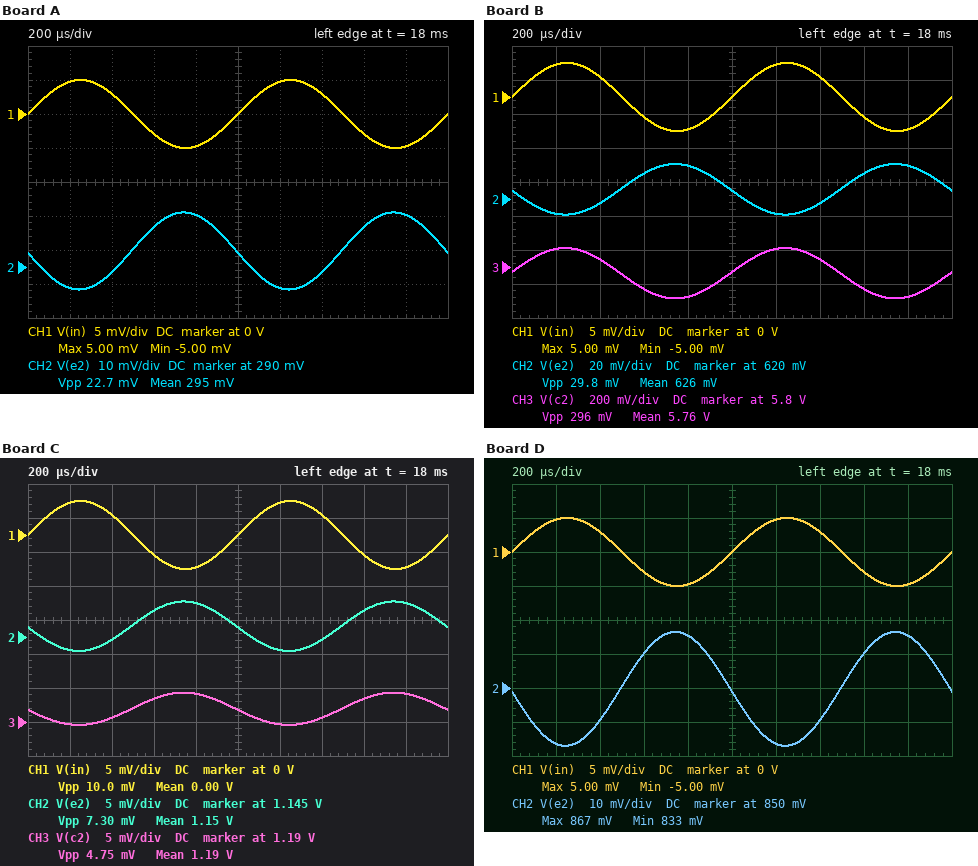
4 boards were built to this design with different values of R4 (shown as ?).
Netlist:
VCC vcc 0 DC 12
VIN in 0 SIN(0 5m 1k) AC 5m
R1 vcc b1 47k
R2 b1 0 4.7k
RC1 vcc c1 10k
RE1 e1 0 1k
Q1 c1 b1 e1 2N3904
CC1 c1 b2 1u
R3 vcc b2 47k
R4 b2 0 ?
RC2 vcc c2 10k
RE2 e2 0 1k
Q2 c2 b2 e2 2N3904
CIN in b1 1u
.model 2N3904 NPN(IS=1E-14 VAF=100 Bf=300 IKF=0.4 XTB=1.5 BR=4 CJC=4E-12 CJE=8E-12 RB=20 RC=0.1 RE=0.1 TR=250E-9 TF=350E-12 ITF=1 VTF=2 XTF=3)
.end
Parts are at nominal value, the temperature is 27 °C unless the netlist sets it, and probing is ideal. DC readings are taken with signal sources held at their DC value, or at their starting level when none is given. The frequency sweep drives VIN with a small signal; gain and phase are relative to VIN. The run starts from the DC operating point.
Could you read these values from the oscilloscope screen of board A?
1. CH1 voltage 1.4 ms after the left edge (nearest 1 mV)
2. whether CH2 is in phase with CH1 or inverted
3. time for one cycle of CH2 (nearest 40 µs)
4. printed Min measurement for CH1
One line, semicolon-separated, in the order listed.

3 mV; inverted; 1.00 ms; -5.00 mV
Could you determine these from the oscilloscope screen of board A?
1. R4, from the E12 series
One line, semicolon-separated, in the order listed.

3.9 kΩ
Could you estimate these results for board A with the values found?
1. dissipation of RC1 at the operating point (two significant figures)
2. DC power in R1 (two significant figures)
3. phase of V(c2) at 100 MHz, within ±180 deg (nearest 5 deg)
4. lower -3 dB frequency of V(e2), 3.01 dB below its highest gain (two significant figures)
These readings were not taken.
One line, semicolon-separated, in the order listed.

2.0 mW; 2.5 mW; 95 deg; 41 Hz
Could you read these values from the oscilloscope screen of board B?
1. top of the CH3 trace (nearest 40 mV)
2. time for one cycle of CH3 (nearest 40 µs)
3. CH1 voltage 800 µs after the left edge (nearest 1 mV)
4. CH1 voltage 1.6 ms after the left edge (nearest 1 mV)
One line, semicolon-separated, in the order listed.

5.92 V; 1.00 ms; -5 mV; -3 mV
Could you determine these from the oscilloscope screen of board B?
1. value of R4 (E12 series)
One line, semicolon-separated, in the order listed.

5.6 kΩ
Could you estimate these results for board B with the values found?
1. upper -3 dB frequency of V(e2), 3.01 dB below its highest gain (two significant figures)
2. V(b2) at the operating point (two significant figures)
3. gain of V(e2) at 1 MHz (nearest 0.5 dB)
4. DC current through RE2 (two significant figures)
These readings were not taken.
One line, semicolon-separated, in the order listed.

1.6 MHz; 1.3 V; 8.0 dB; 630 µA
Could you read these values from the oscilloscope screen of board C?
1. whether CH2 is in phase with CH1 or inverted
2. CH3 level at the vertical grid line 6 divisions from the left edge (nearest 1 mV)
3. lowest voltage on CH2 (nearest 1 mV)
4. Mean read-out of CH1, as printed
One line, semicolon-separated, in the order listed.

inverted; 1.190 V; 1.143 V; 0.00 V
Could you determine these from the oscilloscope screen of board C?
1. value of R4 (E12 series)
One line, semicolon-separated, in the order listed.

12 kΩ
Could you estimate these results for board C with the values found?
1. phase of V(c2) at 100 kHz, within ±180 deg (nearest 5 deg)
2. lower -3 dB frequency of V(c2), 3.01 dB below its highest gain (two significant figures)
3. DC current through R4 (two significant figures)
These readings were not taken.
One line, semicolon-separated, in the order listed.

-170 deg; 440 kHz; 150 µA
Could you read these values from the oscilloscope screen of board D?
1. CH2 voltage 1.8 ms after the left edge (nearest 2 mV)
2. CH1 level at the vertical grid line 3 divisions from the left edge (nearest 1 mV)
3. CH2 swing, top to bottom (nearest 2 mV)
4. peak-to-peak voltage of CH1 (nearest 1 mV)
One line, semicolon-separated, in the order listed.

866 mV; -3 mV; 34 mV; 10 mV
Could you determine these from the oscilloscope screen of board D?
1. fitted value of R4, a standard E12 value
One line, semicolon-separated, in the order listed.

6.8 kΩ
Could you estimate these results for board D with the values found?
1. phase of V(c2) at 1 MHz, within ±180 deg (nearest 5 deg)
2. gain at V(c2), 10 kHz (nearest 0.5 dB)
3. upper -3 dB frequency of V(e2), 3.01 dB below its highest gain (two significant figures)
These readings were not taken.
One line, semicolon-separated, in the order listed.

-45 deg; 30.5 dB; 1.2 MHz
